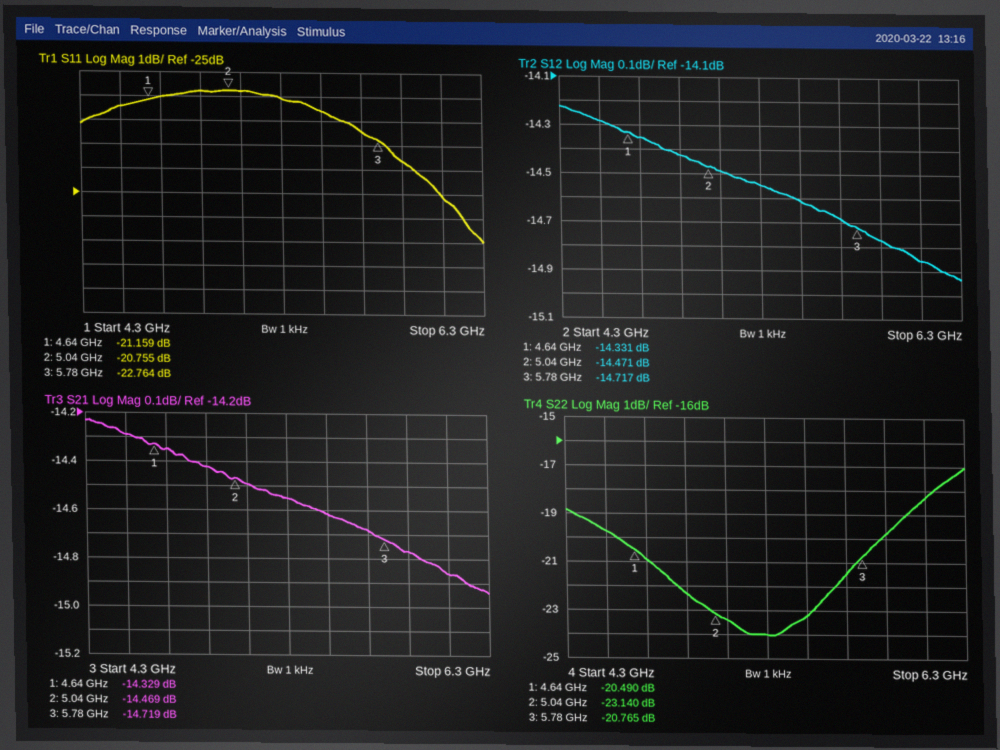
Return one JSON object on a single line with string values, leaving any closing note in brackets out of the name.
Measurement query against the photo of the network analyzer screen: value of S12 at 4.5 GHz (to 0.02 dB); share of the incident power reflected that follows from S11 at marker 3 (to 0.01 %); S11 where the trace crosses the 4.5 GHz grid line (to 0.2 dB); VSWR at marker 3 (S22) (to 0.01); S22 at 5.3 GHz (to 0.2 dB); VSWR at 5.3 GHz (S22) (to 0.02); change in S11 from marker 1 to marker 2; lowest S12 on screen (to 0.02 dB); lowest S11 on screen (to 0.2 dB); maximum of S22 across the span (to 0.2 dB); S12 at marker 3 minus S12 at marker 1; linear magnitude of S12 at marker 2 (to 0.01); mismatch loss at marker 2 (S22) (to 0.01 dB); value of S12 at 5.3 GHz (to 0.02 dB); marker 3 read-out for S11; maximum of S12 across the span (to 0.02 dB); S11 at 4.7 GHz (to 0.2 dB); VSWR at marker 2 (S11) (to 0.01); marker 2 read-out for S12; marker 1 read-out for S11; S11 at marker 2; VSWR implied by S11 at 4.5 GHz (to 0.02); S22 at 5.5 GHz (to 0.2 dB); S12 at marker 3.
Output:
{"value of S12 at 4.5 GHz": "-14.28 dB", "share of the incident power reflected that follows from S11 at marker 3": "0.53 %", "S11 where the trace crosses the 4.5 GHz grid line": "-21.4 dB", "VSWR at marker 3 (S22)": "1.20", "S22 at 5.3 GHz": "-24.0 dB", "VSWR at 5.3 GHz (S22)": "1.14", "change in S11 from marker 1 to marker 2": "0.404 dB", "lowest S12 on screen": "-14.94 dB", "lowest S11 on screen": "-27.0 dB", "maximum of S22 across the span": "-17.0 dB", "S12 at marker 3 minus S12 at marker 1": "-0.386 dB", "linear magnitude of S12 at marker 2": "0.19", "mismatch loss at marker 2 (S22)": "0.02 dB", "value of S12 at 5.3 GHz": "-14.54 dB", "marker 3 read-out for S11": "-22.764 dB", "maximum of S12 across the span": "-14.22 dB", "S11 at 4.7 GHz": "-21.0 dB", "VSWR at marker 2 (S11)": "1.20", "marker 2 read-out for S12": "-14.471 dB", "marker 1 read-out for S11": "-21.159 dB", "S11 at marker 2": "-20.755 dB", "VSWR implied by S11 at 4.5 GHz": "1.18", "S22 at 5.5 GHz": "-23.2 dB", "S12 at marker 3": "-14.717 dB"}
